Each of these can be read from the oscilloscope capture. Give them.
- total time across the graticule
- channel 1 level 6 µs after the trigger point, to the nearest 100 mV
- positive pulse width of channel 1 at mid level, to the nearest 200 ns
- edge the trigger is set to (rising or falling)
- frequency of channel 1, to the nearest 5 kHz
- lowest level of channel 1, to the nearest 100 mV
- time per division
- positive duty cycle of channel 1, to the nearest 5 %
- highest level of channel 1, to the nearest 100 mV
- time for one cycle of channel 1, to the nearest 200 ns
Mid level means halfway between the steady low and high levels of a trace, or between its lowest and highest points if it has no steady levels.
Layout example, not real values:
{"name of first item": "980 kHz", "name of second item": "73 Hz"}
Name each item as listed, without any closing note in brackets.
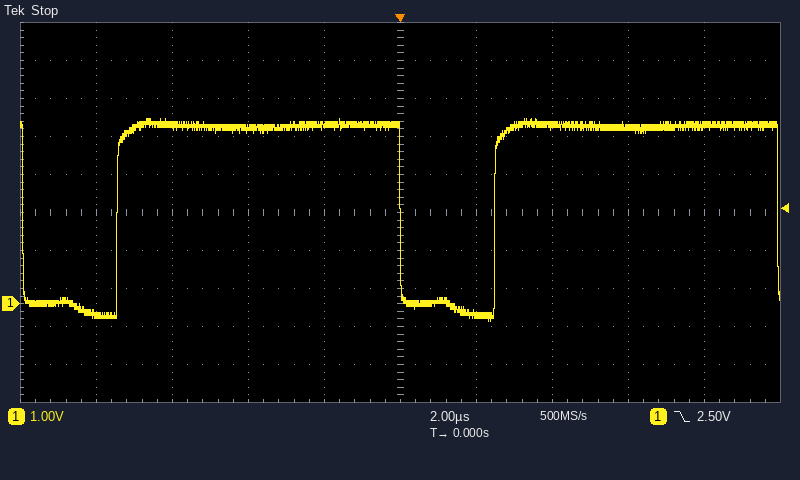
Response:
{"total time across the graticule": "20 µs", "channel 1 level 6 µs after the trigger point, to the nearest 100 mV": "4.6 V", "positive pulse width of channel 1 at mid level, to the nearest 200 ns": "7.4 µs", "edge the trigger is set to": "falling", "frequency of channel 1, to the nearest 5 kHz": "100 kHz", "lowest level of channel 1, to the nearest 100 mV": "-500 mV", "time per division": "2 µs", "positive duty cycle of channel 1, to the nearest 5 %": "75 %", "highest level of channel 1, to the nearest 100 mV": "4.9 V", "time for one cycle of channel 1, to the nearest 200 ns": "10.0 µs"}
